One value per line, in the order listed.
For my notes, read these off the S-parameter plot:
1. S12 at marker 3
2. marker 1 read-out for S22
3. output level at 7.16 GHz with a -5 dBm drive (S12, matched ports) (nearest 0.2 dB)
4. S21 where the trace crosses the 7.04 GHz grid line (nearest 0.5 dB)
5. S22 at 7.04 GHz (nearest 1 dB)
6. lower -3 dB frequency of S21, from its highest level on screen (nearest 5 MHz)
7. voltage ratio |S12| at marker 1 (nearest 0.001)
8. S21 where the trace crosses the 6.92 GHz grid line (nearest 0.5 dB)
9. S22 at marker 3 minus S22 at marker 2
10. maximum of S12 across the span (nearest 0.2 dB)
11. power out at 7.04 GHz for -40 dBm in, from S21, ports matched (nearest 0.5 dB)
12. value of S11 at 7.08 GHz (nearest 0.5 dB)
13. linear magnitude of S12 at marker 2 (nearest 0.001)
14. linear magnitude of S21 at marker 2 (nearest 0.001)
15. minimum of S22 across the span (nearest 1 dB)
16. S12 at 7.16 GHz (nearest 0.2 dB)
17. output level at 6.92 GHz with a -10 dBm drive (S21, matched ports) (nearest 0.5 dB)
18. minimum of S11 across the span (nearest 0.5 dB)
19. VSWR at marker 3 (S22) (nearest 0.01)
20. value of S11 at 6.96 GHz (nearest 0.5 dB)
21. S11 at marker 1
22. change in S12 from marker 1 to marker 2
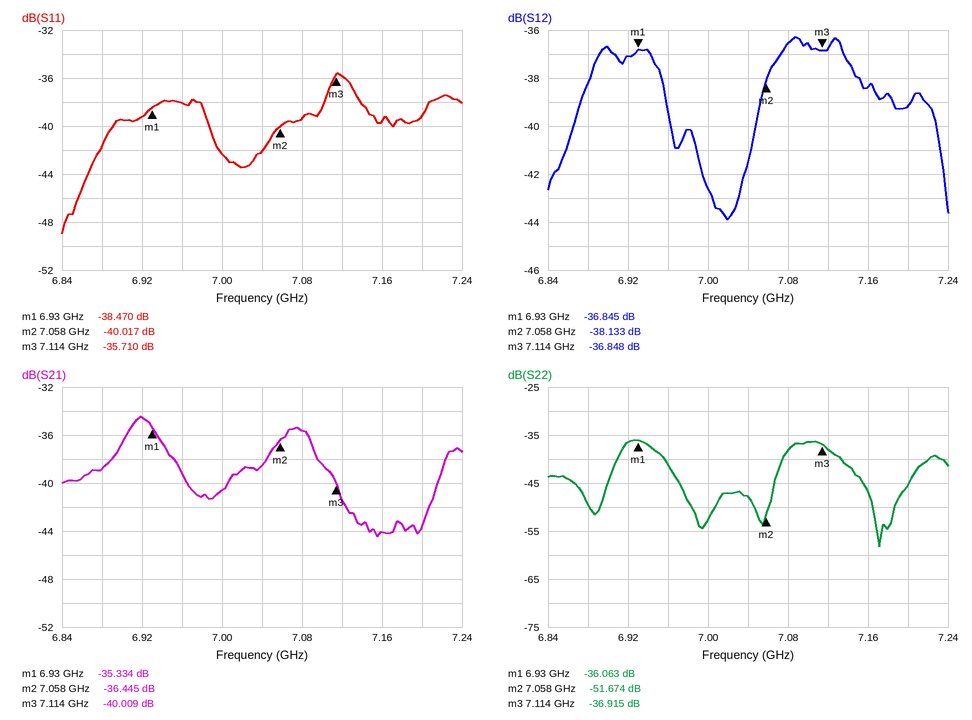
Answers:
-36.848 dB
-36.063 dB
-43.4 dBm
-38.5 dB
-48 dB
6.895 GHz
0.014
-34.5 dB
14.759 dB
-36.2 dB
-78.5 dBm
-39.5 dB
0.012
0.015
-58 dB
-38.4 dB
-44.5 dBm
-49.0 dB
1.03
-38.0 dB
-38.470 dB
-1.288 dB
